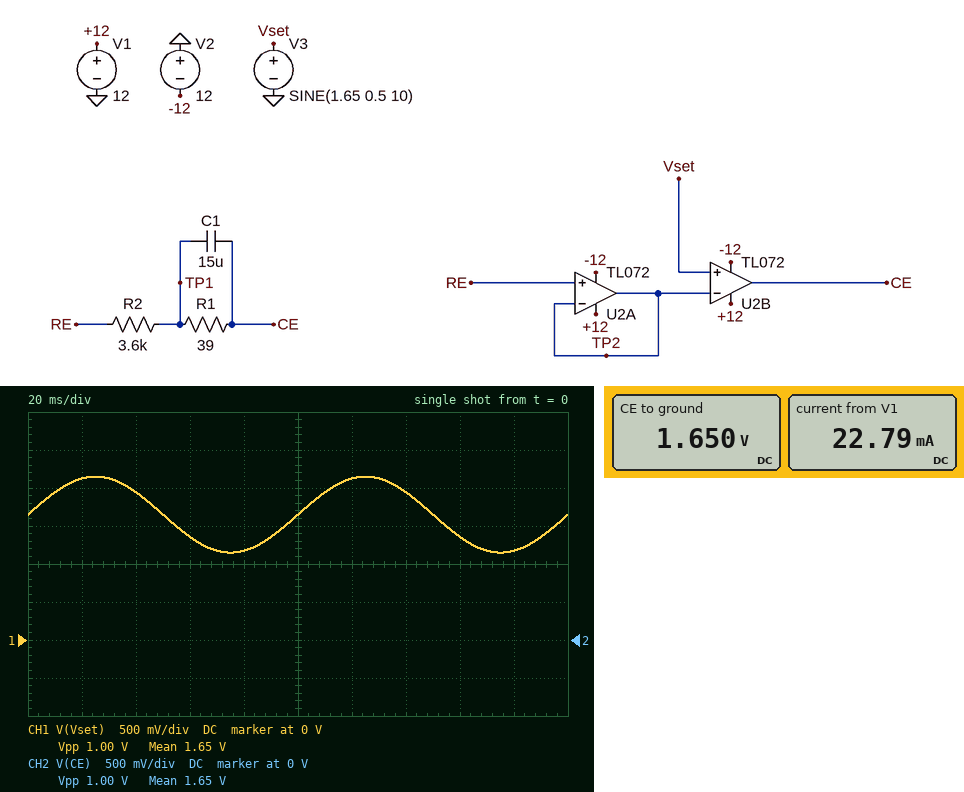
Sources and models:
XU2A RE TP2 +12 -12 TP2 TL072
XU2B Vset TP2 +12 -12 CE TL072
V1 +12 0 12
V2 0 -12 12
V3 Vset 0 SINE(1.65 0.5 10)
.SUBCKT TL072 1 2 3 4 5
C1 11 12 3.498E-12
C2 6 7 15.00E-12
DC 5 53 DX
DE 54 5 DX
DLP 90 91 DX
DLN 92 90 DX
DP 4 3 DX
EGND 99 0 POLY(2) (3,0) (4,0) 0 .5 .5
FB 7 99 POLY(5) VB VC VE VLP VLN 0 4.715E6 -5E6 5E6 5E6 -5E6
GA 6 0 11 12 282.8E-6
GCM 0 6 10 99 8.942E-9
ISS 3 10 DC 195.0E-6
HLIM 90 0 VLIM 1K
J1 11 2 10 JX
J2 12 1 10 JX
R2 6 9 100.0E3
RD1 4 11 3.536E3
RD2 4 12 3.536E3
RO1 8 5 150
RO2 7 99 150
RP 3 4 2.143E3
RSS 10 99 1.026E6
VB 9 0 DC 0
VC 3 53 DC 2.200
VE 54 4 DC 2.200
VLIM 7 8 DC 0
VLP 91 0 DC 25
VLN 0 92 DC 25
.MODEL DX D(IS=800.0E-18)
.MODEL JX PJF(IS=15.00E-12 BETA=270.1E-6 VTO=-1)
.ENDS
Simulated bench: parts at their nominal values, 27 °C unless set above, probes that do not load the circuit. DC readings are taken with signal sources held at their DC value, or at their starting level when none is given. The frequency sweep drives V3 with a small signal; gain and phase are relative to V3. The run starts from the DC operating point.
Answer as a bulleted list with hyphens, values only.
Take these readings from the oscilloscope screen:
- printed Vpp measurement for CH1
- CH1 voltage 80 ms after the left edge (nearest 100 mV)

- 1.00 V
- 1.2 V
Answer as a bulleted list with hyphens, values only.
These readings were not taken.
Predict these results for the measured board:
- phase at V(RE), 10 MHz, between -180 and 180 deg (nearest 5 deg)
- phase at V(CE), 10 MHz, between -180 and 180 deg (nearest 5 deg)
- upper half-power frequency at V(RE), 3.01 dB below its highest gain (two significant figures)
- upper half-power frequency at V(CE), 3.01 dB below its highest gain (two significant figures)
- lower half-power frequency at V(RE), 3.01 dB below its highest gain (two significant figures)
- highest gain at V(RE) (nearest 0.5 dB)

- -150 deg
- -150 deg
- 3.3 MHz
- 3.3 MHz
- 3.0 MHz
- 18.5 dB
